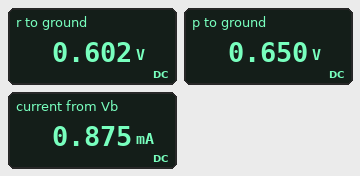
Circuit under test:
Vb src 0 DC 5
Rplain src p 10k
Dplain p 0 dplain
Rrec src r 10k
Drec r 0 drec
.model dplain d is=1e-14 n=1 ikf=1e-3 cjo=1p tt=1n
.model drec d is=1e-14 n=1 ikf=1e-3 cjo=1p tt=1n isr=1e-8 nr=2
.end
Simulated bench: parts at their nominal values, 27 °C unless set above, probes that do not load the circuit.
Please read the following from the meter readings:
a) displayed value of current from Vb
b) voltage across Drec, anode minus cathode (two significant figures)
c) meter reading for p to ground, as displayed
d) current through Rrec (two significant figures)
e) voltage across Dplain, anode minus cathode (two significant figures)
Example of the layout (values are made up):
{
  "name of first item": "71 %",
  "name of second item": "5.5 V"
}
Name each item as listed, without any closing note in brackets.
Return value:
{
  "displayed value of current from Vb": "0.875 mA",
  "voltage across Drec, anode minus cathode": "600 mV",
  "meter reading for p to ground, as displayed": "0.650 V",
  "current through Rrec": "440 µA",
  "voltage across Dplain, anode minus cathode": "650 mV"
}
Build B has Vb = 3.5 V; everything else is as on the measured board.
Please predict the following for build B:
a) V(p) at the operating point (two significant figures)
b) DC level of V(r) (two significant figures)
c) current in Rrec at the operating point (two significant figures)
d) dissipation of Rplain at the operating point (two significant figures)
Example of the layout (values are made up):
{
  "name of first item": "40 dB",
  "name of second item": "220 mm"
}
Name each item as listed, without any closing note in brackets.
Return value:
{
  "V(p) at the operating point": "640 mV",
  "DC level of V(r)": "580 mV",
  "current in Rrec at the operating point": "290 µA",
  "dissipation of Rplain at the operating point": "820 µW"
}
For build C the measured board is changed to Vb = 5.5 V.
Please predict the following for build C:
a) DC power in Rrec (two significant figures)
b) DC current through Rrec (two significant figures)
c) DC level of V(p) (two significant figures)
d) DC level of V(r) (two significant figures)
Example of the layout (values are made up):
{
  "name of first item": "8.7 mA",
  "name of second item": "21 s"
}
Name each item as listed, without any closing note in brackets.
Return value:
{
  "DC power in Rrec": "2.4 mW",
  "DC current through Rrec": "490 µA",
  "DC level of V(p)": "650 mV",
  "DC level of V(r)": "610 mV"
}
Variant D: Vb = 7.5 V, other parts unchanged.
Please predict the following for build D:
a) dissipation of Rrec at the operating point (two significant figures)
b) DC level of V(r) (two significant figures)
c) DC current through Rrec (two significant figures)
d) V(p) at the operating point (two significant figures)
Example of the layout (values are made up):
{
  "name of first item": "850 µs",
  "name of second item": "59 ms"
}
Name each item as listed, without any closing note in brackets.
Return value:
{
  "dissipation of Rrec at the operating point": "4.7 mW",
  "DC level of V(r)": "630 mV",
  "DC current through Rrec": "690 µA",
  "V(p) at the operating point": "670 mV"
}
